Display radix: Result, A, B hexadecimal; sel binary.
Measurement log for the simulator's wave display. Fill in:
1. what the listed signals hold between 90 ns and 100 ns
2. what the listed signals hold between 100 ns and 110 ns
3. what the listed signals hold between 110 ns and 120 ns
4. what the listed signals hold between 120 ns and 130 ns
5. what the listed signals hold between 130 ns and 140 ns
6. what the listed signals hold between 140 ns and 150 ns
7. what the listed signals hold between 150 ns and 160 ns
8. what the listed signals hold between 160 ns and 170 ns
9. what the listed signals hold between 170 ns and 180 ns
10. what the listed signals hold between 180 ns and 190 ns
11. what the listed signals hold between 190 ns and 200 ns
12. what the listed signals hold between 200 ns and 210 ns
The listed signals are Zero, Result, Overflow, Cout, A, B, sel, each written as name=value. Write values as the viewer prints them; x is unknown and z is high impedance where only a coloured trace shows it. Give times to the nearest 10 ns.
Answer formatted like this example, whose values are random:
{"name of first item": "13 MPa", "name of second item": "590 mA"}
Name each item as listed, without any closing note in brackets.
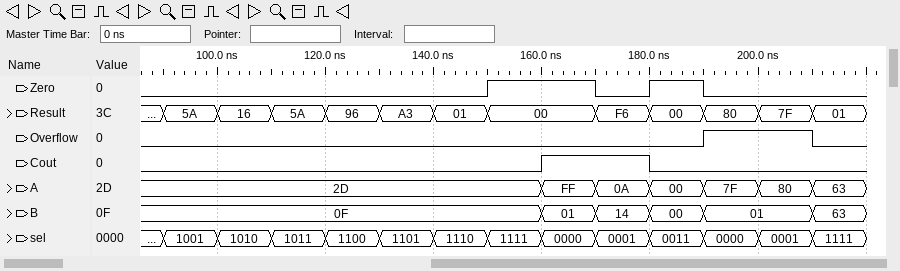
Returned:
{"what the listed signals hold between 90 ns and 100 ns": "Zero=0, Result=5A, Overflow=0, Cout=0, A=2D, B=0F, sel=1001", "what the listed signals hold between 100 ns and 110 ns": "Zero=0, Result=16, Overflow=0, Cout=0, A=2D, B=0F, sel=1010", "what the listed signals hold between 110 ns and 120 ns": "Zero=0, Result=5A, Overflow=0, Cout=0, A=2D, B=0F, sel=1011", "what the listed signals hold between 120 ns and 130 ns": "Zero=0, Result=96, Overflow=0, Cout=0, A=2D, B=0F, sel=1100", "what the listed signals hold between 130 ns and 140 ns": "Zero=0, Result=A3, Overflow=0, Cout=0, A=2D, B=0F, sel=1101", "what the listed signals hold between 140 ns and 150 ns": "Zero=0, Result=01, Overflow=0, Cout=0, A=2D, B=0F, sel=1110", "what the listed signals hold between 150 ns and 160 ns": "Zero=1, Result=00, Overflow=0, Cout=0, A=2D, B=0F, sel=1111", "what the listed signals hold between 160 ns and 170 ns": "Zero=1, Result=00, Overflow=0, Cout=1, A=FF, B=01, sel=0000", "what the listed signals hold between 170 ns and 180 ns": "Zero=0, Result=F6, Overflow=0, Cout=1, A=0A, B=14, sel=0001", "what the listed signals hold between 180 ns and 190 ns": "Zero=1, Result=00, Overflow=0, Cout=0, A=00, B=00, sel=0011", "what the listed signals hold between 190 ns and 200 ns": "Zero=0, Result=80, Overflow=1, Cout=0, A=7F, B=01, sel=0000", "what the listed signals hold between 200 ns and 210 ns": "Zero=0, Result=7F, Overflow=1, Cout=0, A=80, B=01, sel=0001"}
